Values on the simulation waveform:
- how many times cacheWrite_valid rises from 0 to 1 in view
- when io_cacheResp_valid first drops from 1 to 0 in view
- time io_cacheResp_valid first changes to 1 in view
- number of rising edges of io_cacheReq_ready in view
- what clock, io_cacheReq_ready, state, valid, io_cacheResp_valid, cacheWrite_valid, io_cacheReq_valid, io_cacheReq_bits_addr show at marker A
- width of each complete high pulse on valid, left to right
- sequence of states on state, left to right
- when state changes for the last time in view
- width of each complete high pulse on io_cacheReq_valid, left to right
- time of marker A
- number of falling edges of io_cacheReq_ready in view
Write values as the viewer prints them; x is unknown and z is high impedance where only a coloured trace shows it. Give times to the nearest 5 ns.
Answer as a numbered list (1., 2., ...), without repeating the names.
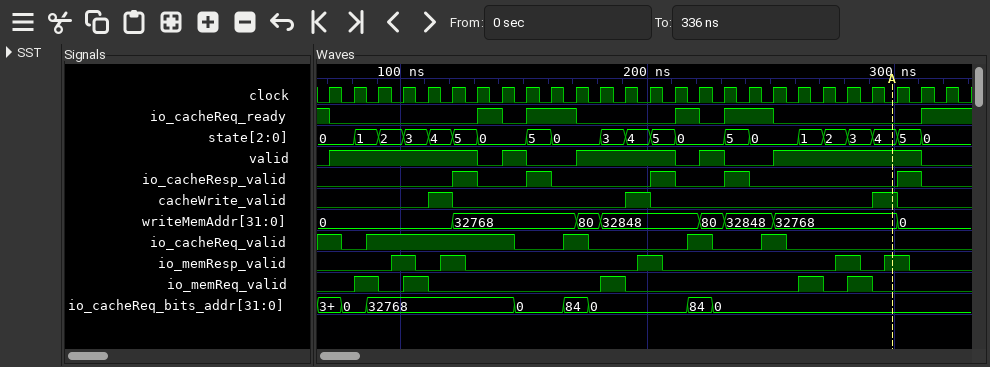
1. 3
2. 130 ns
3. 120 ns
4. 5
5. clock=0, io_cacheReq_ready=0, state=4, valid=1, io_cacheResp_valid=0, cacheWrite_valid=1, io_cacheReq_valid=0, io_cacheReq_bits_addr=0
6. 60 ns, 10 ns, 40 ns, 10 ns, 60 ns
7. 0, 1, 2, 3, 4, 5, 0, 5, 0, 3, 4, 5, 0, 5, 0, 1, 2, 3, 4, 5, 0
8. 310 ns
9. 60 ns, 10 ns, 10 ns, 10 ns
10. 300 ns
11. 5
